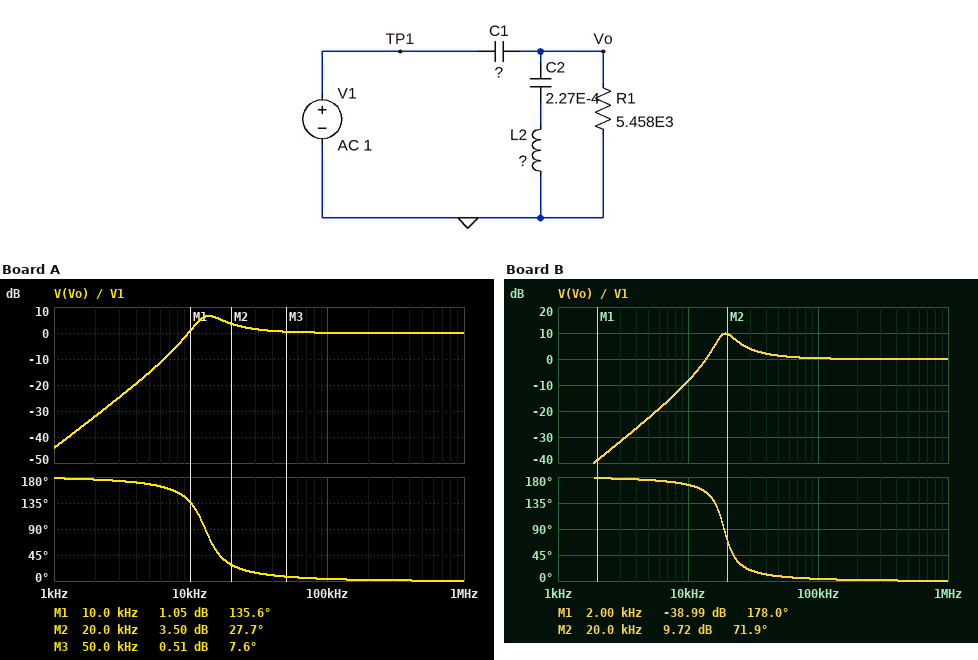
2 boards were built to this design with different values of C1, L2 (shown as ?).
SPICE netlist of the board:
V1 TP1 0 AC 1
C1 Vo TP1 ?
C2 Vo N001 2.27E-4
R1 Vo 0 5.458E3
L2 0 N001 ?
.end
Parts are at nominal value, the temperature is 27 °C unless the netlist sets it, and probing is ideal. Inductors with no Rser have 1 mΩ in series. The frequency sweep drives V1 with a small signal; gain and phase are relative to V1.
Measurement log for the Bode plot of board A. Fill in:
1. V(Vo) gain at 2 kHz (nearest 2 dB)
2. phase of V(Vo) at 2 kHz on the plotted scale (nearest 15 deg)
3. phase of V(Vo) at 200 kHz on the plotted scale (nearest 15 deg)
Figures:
-32 dB
180 deg
0 deg
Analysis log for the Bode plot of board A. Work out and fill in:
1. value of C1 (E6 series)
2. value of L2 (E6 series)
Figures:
4.7 nF
33 mH
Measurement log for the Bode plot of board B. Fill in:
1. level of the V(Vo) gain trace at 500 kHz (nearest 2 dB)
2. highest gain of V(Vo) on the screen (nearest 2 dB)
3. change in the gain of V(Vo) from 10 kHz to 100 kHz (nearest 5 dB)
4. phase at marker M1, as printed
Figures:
0 dB
10 dB
10 dB
178.0 deg
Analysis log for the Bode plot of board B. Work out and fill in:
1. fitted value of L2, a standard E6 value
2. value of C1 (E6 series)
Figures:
15 mH
4.7 nF
